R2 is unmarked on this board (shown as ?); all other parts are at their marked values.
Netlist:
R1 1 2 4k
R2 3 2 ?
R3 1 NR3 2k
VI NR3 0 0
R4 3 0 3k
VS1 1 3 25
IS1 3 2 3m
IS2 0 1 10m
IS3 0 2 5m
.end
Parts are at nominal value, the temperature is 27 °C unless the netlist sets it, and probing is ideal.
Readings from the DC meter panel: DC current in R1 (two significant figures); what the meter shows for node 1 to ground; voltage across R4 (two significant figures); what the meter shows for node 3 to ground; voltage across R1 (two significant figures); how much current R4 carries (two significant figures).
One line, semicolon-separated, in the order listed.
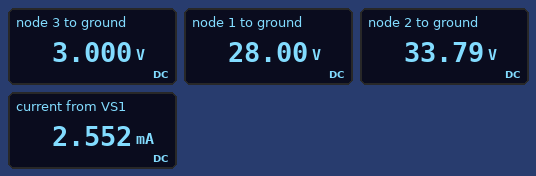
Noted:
1.4 mA; 28.00 V; 3.0 V; 3.000 V; 5.8 V; 1.0 mA
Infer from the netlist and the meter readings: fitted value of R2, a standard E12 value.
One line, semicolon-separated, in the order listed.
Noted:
4.7 kΩ
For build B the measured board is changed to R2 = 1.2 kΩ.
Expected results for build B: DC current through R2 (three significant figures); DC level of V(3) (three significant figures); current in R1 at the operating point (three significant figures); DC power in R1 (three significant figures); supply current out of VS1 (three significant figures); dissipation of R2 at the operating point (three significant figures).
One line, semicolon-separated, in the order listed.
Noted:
11.0 mA; 3.00 V; 2.96 mA; 35.1 mW; 6.96 mA; 144 mW
